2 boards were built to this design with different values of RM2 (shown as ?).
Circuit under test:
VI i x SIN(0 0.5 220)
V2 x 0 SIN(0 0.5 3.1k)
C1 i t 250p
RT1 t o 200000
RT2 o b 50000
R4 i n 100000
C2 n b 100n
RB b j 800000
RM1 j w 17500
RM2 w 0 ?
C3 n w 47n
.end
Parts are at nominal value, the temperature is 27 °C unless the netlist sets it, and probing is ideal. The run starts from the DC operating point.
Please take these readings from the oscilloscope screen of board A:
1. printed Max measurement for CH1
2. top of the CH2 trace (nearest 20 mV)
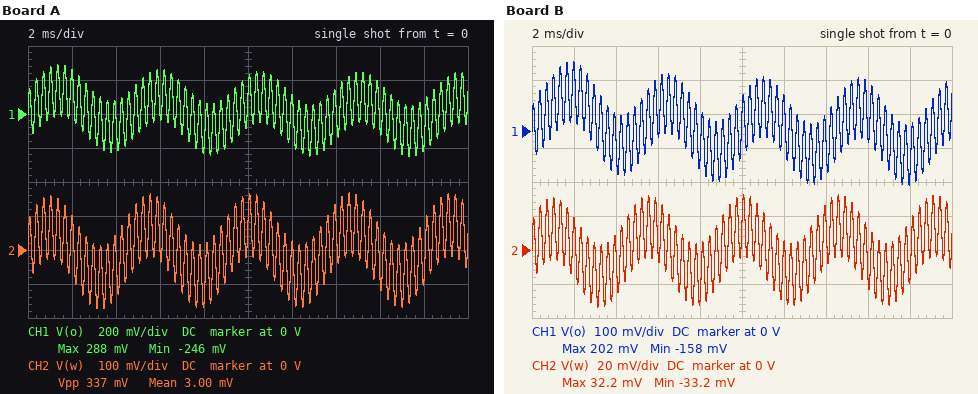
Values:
288 mV
160 mV
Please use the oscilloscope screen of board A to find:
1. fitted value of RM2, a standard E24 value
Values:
18 kΩ
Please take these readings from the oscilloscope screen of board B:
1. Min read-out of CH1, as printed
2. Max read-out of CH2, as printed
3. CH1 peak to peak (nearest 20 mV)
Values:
-158 mV
32.2 mV
360 mV
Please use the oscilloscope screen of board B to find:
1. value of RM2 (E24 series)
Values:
3 kΩ
